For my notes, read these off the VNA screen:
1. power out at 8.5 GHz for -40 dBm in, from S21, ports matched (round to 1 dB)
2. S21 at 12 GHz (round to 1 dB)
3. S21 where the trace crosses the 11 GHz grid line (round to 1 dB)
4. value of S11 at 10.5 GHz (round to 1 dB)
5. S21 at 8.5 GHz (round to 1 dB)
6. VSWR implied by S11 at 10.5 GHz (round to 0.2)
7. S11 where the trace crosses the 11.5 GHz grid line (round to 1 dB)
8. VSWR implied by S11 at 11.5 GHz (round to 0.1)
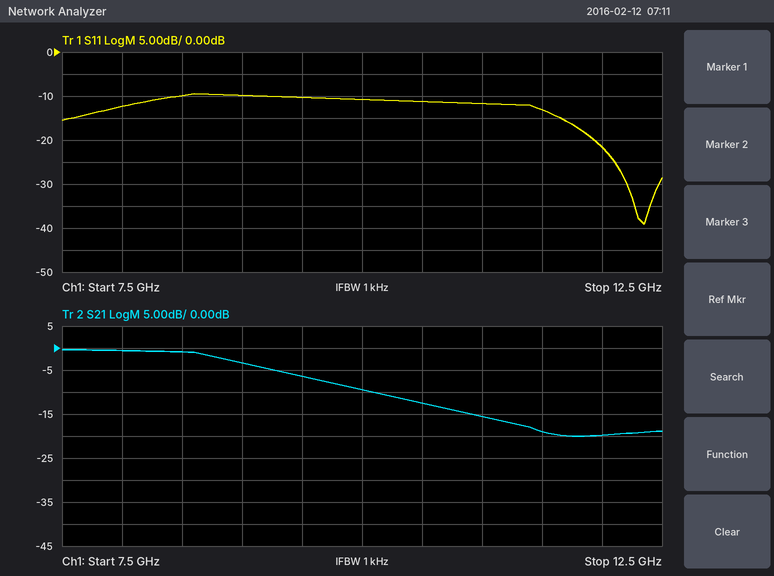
-41 dBm
-20 dB
-16 dB
-11 dB
-1 dB
1.8
-13 dB
1.6
